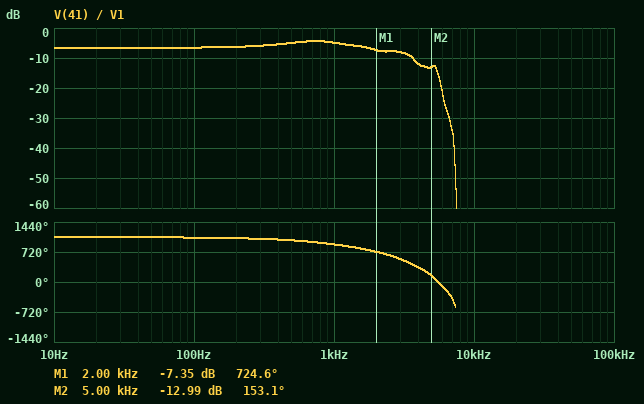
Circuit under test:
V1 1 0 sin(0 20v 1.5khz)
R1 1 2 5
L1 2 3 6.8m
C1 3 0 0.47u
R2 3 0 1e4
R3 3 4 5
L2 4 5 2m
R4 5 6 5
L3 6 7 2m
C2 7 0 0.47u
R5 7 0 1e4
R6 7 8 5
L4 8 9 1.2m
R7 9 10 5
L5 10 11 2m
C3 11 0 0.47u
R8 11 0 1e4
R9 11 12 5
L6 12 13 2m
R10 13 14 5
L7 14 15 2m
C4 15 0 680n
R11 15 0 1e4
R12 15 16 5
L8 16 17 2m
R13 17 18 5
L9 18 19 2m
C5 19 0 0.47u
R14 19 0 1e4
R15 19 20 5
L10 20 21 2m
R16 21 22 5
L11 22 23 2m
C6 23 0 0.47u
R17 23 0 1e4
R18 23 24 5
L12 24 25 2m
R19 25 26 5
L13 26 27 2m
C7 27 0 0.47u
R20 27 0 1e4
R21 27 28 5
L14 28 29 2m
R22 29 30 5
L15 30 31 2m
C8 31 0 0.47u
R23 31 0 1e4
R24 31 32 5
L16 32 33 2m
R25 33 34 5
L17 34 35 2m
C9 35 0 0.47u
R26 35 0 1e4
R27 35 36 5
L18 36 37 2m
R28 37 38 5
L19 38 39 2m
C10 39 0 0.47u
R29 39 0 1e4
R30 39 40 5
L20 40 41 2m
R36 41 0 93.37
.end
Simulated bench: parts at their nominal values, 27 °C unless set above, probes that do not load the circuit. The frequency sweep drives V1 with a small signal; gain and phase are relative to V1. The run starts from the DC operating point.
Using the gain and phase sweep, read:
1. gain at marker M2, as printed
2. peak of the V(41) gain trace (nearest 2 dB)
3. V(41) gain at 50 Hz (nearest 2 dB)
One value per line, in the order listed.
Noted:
-12.99 dB
-4 dB
-6 dB
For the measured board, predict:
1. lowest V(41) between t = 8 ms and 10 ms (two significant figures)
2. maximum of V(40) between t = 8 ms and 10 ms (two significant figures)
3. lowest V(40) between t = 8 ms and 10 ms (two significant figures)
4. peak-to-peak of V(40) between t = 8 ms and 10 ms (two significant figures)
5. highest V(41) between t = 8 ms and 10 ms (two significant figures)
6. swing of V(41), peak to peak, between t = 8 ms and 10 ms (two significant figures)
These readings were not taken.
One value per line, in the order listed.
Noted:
-10 V
10 V
-10 V
20 V
10 V
20 V
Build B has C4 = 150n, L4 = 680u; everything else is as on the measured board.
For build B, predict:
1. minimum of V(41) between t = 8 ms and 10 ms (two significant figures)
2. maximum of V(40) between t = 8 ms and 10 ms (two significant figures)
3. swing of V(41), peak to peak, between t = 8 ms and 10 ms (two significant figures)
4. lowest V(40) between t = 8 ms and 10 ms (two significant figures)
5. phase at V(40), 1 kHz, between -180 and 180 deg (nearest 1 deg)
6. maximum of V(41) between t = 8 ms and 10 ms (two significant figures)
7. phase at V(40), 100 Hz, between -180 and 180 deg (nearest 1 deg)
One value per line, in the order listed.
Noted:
-11 V
12 V
23 V
-12 V
-155 deg
11 V
-13 deg
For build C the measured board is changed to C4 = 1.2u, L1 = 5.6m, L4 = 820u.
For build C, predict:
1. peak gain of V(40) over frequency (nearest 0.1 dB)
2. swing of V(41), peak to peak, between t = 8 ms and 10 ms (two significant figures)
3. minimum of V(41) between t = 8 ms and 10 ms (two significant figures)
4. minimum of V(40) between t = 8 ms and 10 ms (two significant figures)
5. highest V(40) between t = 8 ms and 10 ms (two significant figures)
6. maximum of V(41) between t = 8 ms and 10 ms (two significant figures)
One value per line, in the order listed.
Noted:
-4.1 dB
18 V
-8.9 V
-9.1 V
9.1 V
8.9 V
